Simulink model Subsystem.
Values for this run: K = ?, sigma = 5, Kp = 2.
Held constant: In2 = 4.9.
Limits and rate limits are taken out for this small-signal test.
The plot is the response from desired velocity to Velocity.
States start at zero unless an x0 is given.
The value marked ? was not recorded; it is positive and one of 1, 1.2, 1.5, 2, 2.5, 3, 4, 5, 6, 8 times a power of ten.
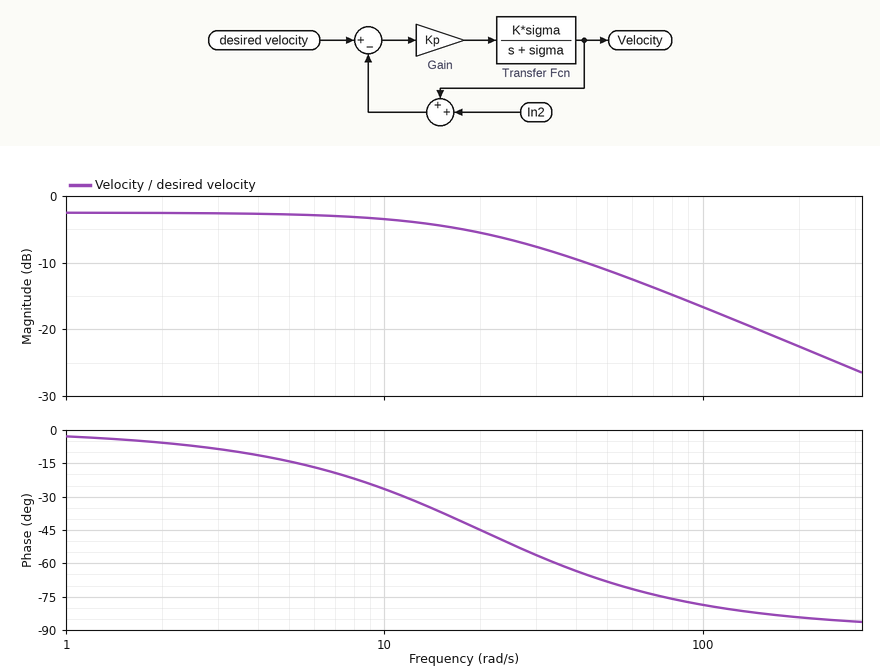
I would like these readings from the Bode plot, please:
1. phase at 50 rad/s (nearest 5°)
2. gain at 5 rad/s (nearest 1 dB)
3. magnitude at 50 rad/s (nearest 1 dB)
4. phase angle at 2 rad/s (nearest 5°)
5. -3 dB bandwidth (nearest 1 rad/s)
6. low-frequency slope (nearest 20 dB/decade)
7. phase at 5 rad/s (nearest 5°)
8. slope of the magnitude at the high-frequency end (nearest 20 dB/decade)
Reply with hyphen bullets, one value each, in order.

- -70°
- -3 dB
- -11 dB
- -5°
- 20 rad/s
- 0 dB/decade
- -15°
- -20 dB/decade
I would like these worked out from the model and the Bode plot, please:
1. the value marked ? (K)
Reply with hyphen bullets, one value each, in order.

- 1.5
